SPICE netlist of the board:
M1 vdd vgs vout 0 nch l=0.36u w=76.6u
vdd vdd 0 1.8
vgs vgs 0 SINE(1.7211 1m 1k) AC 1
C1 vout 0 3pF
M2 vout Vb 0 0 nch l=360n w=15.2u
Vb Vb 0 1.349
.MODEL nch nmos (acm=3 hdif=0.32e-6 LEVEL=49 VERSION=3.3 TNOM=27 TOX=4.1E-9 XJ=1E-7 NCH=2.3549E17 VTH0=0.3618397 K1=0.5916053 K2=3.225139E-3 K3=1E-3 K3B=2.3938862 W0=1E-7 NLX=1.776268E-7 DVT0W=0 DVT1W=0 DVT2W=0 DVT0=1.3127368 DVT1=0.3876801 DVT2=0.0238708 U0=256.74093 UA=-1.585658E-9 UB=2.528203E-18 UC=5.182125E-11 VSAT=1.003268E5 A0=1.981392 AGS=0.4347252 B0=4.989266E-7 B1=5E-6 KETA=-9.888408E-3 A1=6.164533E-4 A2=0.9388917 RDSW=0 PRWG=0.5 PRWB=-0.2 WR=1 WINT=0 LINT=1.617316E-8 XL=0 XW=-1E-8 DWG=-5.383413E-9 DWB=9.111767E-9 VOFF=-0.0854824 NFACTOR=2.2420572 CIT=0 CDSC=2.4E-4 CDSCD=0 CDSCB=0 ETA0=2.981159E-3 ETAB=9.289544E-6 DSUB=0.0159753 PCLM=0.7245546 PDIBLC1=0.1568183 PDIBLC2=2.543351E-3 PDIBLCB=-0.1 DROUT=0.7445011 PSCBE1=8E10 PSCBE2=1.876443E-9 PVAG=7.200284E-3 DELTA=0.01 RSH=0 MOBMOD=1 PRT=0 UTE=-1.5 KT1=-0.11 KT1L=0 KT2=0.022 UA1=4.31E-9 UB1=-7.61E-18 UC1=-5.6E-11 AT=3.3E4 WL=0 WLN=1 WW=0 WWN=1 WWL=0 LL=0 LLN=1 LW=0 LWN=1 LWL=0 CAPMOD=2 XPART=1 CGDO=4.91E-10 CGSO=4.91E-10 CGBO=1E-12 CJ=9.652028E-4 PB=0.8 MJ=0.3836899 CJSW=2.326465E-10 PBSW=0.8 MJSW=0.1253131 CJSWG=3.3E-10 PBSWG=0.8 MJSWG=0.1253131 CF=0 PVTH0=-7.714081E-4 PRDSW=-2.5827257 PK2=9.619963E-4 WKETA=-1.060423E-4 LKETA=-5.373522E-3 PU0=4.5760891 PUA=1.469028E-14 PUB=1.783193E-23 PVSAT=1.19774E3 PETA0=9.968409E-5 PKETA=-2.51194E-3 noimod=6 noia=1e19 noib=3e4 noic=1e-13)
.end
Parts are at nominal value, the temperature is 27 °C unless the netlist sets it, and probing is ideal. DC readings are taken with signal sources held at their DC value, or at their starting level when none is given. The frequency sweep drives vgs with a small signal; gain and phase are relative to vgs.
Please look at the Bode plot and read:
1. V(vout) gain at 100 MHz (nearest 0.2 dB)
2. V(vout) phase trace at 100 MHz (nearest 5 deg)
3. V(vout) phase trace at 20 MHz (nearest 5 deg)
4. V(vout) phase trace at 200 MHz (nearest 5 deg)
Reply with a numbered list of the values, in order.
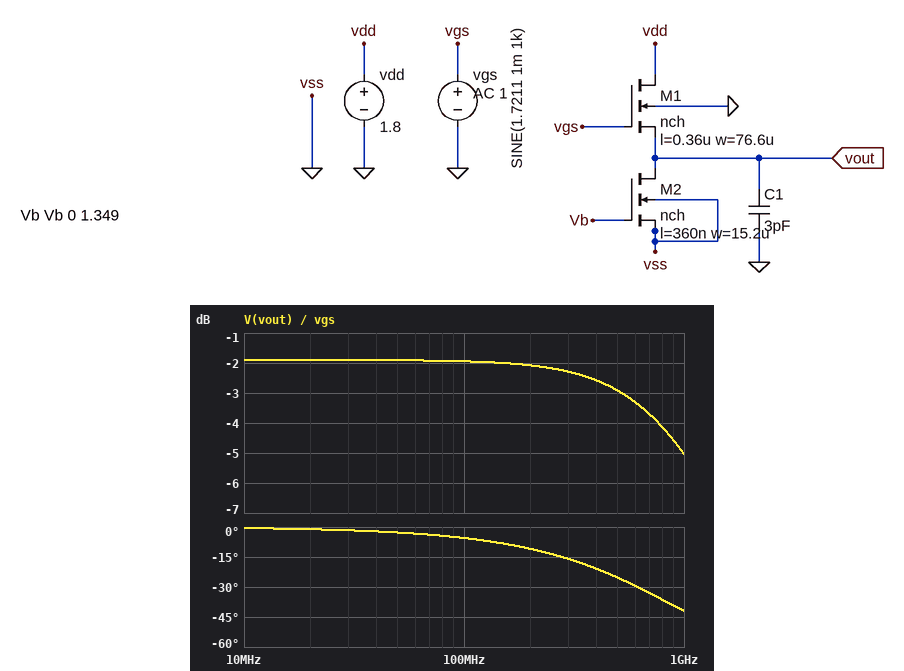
1. -2.0 dB
2. -5 deg
3. 0 deg
4. -10 deg
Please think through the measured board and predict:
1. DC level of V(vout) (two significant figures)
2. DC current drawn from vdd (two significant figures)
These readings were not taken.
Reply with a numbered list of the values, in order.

1. 750 mV
2. 3.0 mA
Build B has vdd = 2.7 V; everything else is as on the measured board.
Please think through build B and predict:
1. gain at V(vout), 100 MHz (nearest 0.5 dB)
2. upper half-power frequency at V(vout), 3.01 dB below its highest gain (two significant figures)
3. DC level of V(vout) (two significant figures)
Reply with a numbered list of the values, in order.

1. -2.0 dB
2. 980 MHz
3. 760 mV
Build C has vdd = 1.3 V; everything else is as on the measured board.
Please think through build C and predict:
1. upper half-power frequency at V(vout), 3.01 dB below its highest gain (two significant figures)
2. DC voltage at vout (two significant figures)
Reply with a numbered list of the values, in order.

1. 960 MHz
2. 740 mV
